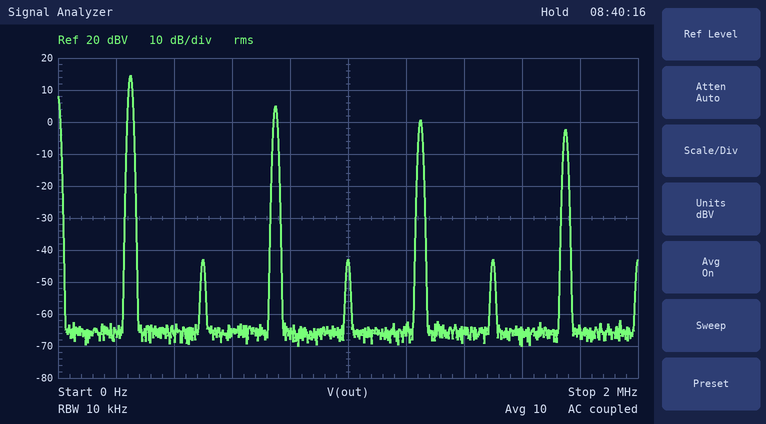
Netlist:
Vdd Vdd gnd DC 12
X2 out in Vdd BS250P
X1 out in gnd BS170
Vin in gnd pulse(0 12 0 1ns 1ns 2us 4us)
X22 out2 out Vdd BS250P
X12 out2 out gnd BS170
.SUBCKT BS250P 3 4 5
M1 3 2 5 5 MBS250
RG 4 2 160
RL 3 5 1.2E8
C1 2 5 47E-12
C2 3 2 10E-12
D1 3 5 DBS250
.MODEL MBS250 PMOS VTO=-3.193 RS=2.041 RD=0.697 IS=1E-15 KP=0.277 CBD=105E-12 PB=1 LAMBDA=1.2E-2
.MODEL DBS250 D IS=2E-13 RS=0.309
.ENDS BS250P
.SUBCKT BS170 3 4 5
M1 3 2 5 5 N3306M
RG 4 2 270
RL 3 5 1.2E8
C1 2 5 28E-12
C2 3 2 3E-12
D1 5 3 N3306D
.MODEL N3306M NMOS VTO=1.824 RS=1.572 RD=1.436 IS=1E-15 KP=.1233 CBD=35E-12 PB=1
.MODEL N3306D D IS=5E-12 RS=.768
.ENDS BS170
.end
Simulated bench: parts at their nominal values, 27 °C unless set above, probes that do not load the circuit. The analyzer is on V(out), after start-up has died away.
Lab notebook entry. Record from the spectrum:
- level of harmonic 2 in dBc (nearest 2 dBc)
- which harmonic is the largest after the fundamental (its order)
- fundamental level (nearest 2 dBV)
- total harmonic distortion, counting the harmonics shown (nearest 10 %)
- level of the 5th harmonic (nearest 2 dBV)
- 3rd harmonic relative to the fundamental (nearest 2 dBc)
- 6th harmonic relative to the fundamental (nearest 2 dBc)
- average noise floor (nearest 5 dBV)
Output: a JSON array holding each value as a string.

["-58 dBc", "3", "14 dBV", "40 %", "0 dBV", "-10 dBc", "-58 dBc", "-65 dBV"]
